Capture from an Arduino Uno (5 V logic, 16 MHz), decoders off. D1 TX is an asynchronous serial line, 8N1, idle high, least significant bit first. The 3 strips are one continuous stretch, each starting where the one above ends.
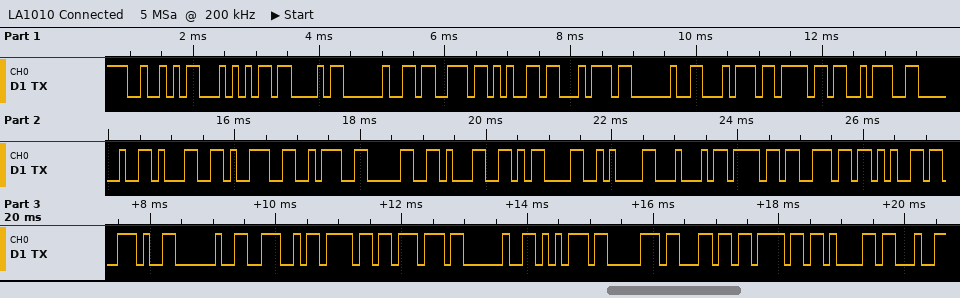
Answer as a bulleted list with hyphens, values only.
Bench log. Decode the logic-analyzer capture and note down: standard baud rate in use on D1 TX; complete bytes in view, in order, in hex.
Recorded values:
- 9600 baud
- 52 54 43 20 73 65 74 20 74 6F 3A 20 31 39 3A 30 31 0D 0A 44 6F 6E 65 2E 20 4E 6F 77 20 75 70 6C 6F 61
